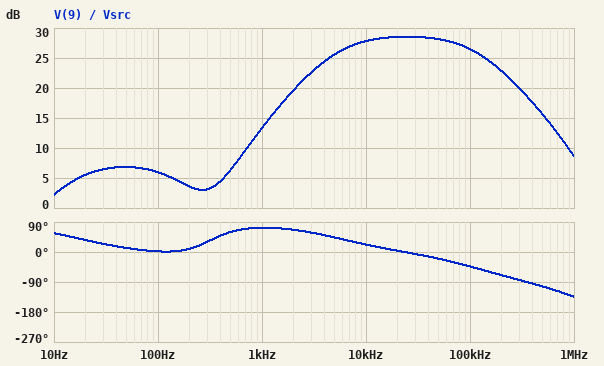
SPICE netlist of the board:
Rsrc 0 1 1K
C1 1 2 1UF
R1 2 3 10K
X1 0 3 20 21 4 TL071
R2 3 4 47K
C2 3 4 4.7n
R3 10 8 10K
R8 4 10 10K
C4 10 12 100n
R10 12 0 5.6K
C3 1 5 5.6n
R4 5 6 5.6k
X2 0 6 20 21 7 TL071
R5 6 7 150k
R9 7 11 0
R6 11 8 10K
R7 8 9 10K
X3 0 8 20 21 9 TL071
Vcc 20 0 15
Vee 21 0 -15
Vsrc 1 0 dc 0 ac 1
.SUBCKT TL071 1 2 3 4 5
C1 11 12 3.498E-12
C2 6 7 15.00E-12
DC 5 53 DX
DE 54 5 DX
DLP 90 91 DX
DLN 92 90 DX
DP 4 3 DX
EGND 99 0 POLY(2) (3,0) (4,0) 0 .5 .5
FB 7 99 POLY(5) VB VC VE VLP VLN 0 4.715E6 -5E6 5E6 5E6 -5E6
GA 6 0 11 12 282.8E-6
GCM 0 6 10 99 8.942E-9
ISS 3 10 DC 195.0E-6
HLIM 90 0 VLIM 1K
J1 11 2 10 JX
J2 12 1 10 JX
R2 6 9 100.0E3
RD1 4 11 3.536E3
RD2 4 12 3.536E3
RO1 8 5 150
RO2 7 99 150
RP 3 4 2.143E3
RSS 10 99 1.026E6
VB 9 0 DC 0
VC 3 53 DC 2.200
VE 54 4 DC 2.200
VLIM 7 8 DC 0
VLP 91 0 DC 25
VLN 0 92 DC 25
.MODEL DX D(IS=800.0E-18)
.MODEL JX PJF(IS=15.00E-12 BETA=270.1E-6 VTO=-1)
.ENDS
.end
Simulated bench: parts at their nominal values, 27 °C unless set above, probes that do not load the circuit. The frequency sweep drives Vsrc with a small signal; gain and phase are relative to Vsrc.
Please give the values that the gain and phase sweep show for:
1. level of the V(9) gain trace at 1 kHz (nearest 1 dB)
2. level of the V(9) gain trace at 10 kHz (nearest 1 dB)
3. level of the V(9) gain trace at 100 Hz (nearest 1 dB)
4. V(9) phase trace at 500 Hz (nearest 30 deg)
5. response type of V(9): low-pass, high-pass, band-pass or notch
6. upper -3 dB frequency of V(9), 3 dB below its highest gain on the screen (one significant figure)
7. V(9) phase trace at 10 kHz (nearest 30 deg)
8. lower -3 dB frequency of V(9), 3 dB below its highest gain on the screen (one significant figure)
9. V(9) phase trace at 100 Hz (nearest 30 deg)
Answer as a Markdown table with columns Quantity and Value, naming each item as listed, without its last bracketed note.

| Quantity | Value |
|---|---|
| level of the V(9) gain trace at 1 kHz | 13 dB |
| level of the V(9) gain trace at 10 kHz | 28 dB |
| level of the V(9) gain trace at 100 Hz | 6 dB |
| V(9) phase trace at 500 Hz | 60 deg |
| response type of V(9): low-pass, high-pass, band-pass or notch | band-pass |
| upper -3 dB frequency of V(9), 3 dB below its highest gain on the screen | 100 kHz |
| V(9) phase trace at 10 kHz | 30 deg |
| lower -3 dB frequency of V(9), 3 dB below its highest gain on the screen | 5 kHz |
| V(9) phase trace at 100 Hz | 0 deg |
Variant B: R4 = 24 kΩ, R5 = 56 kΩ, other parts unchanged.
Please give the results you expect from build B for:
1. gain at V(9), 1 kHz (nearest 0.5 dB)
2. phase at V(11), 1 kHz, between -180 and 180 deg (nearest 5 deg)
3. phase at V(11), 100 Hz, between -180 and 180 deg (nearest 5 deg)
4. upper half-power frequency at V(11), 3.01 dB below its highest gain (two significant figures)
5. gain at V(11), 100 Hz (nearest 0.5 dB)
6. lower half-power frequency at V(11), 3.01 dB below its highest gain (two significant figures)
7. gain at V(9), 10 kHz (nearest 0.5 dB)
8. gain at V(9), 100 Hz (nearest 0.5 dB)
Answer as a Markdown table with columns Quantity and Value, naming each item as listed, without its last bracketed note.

| Quantity | Value |
|---|---|
| gain at V(9), 1 kHz | 3.0 dB |
| phase at V(11), 1 kHz, between -180 and 180 deg | -130 deg |
| phase at V(11), 100 Hz, between -180 and 180 deg | -95 deg |
| upper half-power frequency at V(11), 3.01 dB below its highest gain | 1.2 MHz |
| gain at V(11), 100 Hz | -14.0 dB |
| lower half-power frequency at V(11), 3.01 dB below its highest gain | 1.2 kHz |
| gain at V(9), 10 kHz | 7.5 dB |
| gain at V(9), 100 Hz | 6.0 dB |
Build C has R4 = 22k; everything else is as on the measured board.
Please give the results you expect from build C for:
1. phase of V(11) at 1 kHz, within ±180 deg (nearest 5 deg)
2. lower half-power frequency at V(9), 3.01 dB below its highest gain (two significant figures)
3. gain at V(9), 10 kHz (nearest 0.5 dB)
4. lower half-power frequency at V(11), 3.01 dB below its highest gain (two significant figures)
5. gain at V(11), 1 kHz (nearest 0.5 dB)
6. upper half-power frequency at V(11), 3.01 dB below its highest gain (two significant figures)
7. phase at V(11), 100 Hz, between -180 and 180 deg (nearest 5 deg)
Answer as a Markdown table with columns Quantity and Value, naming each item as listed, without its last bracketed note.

| Quantity | Value |
|---|---|
| phase of V(11) at 1 kHz, within ±180 deg | -130 deg |
| lower half-power frequency at V(9), 3.01 dB below its highest gain | 1.4 kHz |
| gain at V(9), 10 kHz | 16.5 dB |
| lower half-power frequency at V(11), 3.01 dB below its highest gain | 1.3 kHz |
| gain at V(11), 1 kHz | 12.5 dB |
| upper half-power frequency at V(11), 3.01 dB below its highest gain | 450 kHz |
| phase at V(11), 100 Hz, between -180 and 180 deg | -95 deg |
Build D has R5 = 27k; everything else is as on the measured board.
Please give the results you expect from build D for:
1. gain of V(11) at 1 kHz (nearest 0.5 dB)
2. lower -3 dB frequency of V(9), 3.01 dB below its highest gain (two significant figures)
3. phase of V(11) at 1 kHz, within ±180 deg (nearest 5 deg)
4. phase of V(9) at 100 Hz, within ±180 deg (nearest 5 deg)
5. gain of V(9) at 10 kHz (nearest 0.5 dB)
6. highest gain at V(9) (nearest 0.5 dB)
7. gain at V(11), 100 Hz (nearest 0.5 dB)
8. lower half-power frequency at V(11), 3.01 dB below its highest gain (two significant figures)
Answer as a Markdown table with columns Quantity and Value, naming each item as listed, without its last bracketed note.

| Quantity | Value |
|---|---|
| gain of V(11) at 1 kHz | -0.5 dB |
| lower -3 dB frequency of V(9), 3.01 dB below its highest gain | 5.3 kHz |
| phase of V(11) at 1 kHz, within ±180 deg | -100 deg |
| phase of V(9) at 100 Hz, within ±180 deg | -10 deg |
| gain of V(9) at 10 kHz | 12.5 dB |
| highest gain at V(9) | 13.5 dB |
| gain at V(11), 100 Hz | -20.5 dB |
| lower half-power frequency at V(11), 3.01 dB below its highest gain | 5.0 kHz |
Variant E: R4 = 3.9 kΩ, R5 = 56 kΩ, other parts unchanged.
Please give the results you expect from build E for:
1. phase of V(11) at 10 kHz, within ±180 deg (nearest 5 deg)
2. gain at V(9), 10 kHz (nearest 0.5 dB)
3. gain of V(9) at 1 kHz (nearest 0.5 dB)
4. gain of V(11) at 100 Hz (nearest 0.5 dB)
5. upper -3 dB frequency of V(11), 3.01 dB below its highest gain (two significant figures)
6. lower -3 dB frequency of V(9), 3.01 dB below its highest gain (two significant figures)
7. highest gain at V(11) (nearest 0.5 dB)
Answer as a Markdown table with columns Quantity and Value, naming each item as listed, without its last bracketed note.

| Quantity | Value |
|---|---|
| phase of V(11) at 10 kHz, within ±180 deg | -145 deg |
| gain at V(9), 10 kHz | 21.5 dB |
| gain of V(9) at 1 kHz | 3.0 dB |
| gain of V(11) at 100 Hz | -14.0 dB |
| upper -3 dB frequency of V(11), 3.01 dB below its highest gain | 230 kHz |
| lower -3 dB frequency of V(9), 3.01 dB below its highest gain | 7.2 kHz |
| highest gain at V(11) | 23.0 dB |
